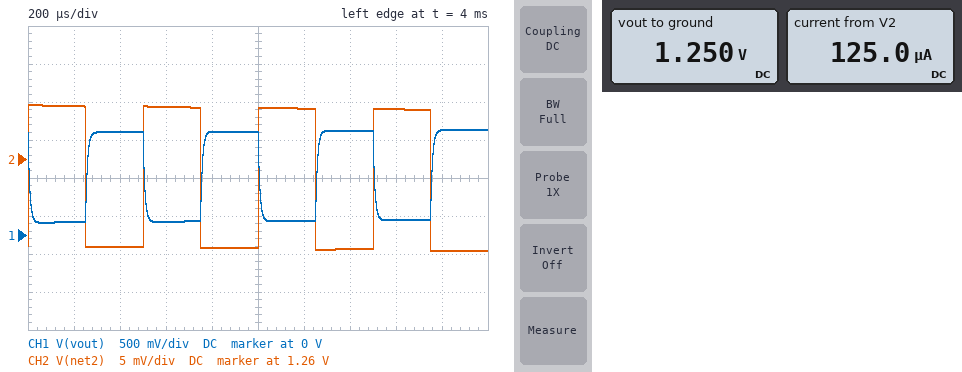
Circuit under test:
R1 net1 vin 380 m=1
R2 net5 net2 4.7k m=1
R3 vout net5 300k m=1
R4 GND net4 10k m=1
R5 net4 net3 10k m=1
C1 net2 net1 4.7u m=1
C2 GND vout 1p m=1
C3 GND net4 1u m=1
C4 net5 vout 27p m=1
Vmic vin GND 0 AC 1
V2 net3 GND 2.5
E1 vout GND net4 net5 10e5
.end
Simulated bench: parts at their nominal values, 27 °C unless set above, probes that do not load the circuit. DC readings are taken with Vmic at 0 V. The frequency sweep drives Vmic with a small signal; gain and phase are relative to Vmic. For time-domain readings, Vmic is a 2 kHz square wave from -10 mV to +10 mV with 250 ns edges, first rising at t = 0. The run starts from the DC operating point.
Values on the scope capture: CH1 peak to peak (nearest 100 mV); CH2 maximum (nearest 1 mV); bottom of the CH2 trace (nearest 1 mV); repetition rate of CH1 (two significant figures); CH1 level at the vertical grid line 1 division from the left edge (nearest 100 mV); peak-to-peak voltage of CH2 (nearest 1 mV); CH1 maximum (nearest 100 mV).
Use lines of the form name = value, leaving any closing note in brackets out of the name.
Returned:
CH1 peak to peak = 1.2 V
CH2 maximum = 1.267 V
bottom of the CH2 trace = 1.248 V
repetition rate of CH1 = 2.0 kHz
CH1 level at the vertical grid line 1 division from the left edge = 200 mV
peak-to-peak voltage of CH2 = 19 mV
CH1 maximum = 1.4 V
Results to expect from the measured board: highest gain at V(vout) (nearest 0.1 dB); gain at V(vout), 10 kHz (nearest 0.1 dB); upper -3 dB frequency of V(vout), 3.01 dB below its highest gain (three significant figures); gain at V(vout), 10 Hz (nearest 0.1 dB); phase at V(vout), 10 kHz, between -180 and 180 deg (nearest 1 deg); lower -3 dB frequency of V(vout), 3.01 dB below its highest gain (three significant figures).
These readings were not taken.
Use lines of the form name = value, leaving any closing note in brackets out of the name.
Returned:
highest gain at V(vout) = 35.4 dB
gain at V(vout), 10 kHz = 34.4 dB
upper -3 dB frequency of V(vout), 3.01 dB below its highest gain = 19.7 kHz
gain at V(vout), 10 Hz = 33.8 dB
phase at V(vout), 10 kHz, between -180 and 180 deg = 153 deg
lower -3 dB frequency of V(vout), 3.01 dB below its highest gain = 6.66 Hz
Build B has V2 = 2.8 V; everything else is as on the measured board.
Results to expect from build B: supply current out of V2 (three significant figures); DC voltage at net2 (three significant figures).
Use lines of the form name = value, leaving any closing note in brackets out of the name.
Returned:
supply current out of V2 = 140 µA
DC voltage at net2 = 1.40 V
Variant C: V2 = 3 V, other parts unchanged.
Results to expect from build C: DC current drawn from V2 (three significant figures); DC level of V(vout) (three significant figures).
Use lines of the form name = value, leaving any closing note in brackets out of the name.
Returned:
DC current drawn from V2 = 150 µA
DC level of V(vout) = 1.50 V
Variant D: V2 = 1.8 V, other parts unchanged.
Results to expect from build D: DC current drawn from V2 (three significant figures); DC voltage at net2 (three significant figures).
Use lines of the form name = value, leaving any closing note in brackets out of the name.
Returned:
DC current drawn from V2 = 90.0 µA
DC voltage at net2 = 900 mV
